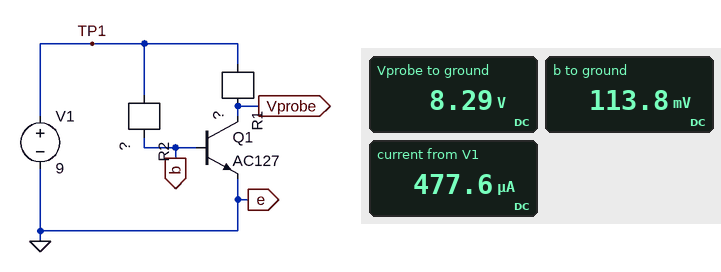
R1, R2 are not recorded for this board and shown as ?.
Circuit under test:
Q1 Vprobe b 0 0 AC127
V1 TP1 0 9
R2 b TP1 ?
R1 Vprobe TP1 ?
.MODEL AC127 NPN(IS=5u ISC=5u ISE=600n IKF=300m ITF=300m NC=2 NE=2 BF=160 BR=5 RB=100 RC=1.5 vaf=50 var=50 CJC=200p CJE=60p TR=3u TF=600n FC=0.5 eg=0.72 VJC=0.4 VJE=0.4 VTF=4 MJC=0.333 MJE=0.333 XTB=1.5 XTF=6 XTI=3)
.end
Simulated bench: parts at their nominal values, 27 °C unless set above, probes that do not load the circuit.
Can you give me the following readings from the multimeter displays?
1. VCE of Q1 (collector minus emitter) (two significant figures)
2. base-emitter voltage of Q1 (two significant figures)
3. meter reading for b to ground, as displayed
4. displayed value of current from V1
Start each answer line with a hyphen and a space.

- 8.3 V
- 110 mV
- 113.8 mV
- 477.6 µA
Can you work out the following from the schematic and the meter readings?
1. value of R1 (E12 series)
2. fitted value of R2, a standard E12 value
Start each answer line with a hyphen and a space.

- 1.5 kΩ
- 6.8 MΩ
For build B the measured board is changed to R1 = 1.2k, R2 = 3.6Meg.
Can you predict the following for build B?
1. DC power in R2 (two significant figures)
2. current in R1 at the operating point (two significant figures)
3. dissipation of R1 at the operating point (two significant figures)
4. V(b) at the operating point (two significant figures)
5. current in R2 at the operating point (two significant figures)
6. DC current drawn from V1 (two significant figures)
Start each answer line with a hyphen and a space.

- 22 µW
- 580 µA
- 410 µW
- 120 mV
- 2.5 µA
- 590 µA
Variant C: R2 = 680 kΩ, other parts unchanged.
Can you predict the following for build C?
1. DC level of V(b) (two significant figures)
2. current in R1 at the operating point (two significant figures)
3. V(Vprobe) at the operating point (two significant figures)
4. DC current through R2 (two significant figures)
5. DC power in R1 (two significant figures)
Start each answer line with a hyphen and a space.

- 150 mV
- 1.7 mA
- 6.5 V
- 13 µA
- 4.2 mW
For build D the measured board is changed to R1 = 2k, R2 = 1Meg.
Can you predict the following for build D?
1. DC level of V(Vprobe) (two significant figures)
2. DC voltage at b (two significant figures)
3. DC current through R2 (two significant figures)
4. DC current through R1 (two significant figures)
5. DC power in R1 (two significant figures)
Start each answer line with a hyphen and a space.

- 6.6 V
- 140 mV
- 8.9 µA
- 1.2 mA
- 2.9 mW
